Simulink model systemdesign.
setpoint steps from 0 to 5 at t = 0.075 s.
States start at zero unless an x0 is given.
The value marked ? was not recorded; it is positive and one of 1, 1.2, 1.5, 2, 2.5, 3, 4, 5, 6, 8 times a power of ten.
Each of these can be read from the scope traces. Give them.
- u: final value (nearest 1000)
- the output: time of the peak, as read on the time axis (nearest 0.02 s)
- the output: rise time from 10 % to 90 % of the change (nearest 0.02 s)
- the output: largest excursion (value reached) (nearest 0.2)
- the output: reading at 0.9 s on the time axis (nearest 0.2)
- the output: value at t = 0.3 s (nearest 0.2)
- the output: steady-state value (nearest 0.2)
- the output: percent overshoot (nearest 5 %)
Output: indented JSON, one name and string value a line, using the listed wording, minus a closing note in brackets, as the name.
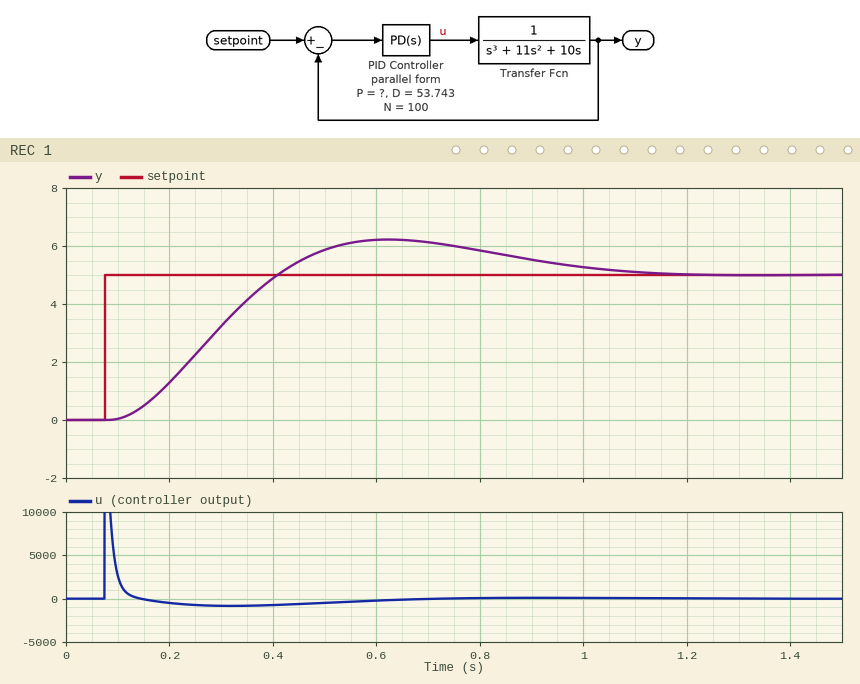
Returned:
{
  "u: final value": "0",
  "the output: time of the peak, as read on the time axis": "0.62 s",
  "the output: rise time from 10 % to 90 % of the change": "0.22 s",
  "the output: largest excursion (value reached)": "6.2",
  "the output: reading at 0.9 s on the time axis": "5.6",
  "the output: value at t = 0.3 s": "3.2",
  "the output: steady-state value": "5.0",
  "the output: percent overshoot": "25 %"
}
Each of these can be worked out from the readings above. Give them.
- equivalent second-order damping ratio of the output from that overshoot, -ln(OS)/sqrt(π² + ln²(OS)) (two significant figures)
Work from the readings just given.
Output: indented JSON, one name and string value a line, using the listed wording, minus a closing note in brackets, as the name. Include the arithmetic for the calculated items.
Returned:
{
  "equivalent second-order damping ratio of the output from that overshoot, -ln(OS)/sqrt(π² + ln²(OS))": "ln(0.25) = -1.386; 1.386 / sqrt(9.870 + 1.922) = 0.40"
}
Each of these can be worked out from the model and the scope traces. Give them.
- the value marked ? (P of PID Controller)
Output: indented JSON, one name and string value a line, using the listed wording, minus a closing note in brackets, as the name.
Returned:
{
  "the value marked ?": "120"
}
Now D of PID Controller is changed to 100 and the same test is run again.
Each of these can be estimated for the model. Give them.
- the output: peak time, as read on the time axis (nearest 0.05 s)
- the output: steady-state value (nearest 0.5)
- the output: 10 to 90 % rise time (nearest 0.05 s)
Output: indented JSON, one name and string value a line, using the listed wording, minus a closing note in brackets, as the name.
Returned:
{
  "the output: peak time, as read on the time axis": "0.45 s",
  "the output: steady-state value": "5.0",
  "the output: 10 to 90 % rise time": "0.15 s"
}
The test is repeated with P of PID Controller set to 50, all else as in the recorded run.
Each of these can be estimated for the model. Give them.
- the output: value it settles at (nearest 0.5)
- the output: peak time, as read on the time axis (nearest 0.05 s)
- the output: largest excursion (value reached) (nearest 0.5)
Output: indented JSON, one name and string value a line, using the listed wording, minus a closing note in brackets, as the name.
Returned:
{
  "the output: value it settles at": "5.0",
  "the output: peak time, as read on the time axis": "0.65 s",
  "the output: largest excursion (value reached)": "5.5"
}
